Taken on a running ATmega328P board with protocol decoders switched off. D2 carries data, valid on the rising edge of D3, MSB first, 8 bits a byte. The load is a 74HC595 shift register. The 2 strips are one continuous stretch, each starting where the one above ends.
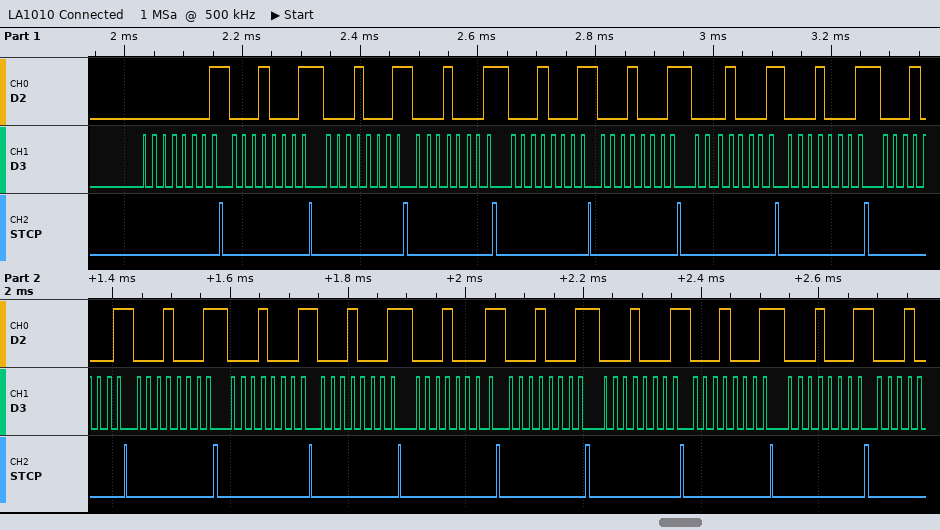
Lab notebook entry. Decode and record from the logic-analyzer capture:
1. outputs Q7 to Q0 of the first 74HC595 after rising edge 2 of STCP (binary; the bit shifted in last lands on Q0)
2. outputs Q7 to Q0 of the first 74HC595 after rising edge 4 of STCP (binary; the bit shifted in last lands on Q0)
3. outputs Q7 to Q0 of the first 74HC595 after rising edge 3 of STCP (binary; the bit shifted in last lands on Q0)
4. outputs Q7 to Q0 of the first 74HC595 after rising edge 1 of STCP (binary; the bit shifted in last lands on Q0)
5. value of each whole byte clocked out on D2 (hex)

00010001
00010001
00010001
00000001
01 11 11 11 11 11 11 11 11 11 11 11 11 11 11 11 11
